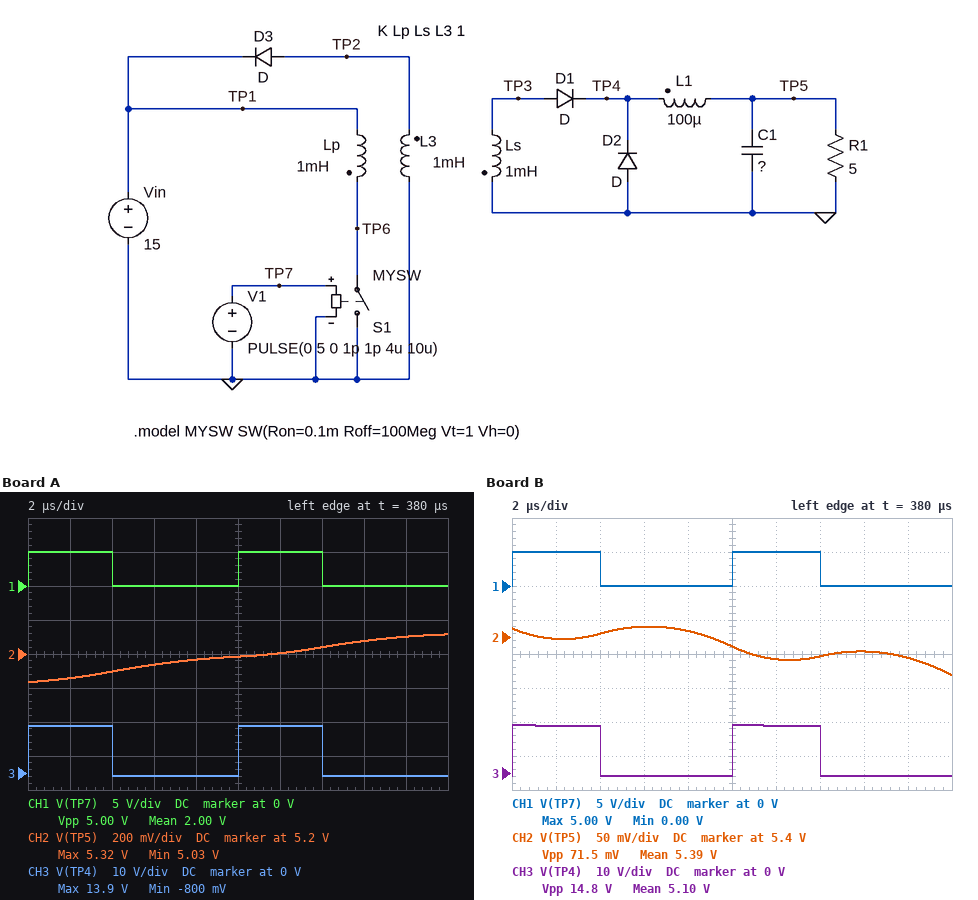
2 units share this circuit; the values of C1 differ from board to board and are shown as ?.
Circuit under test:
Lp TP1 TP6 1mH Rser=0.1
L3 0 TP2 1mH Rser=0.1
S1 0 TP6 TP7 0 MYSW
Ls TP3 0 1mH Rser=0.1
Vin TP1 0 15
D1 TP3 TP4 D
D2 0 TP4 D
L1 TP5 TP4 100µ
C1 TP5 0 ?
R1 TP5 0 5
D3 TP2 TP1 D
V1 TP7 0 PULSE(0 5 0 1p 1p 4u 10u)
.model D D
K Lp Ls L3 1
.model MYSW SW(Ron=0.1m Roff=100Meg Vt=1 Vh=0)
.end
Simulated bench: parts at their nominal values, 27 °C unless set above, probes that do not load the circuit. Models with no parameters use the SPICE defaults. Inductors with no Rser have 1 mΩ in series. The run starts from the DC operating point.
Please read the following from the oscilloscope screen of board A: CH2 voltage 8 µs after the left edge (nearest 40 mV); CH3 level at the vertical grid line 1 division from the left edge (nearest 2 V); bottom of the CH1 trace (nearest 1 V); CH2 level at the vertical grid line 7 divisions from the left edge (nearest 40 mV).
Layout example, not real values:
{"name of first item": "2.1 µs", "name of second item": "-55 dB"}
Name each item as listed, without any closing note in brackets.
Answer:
{"CH2 voltage 8 µs after the left edge": "5.16 V", "CH3 level at the vertical grid line 1 division from the left edge": "14 V", "bottom of the CH1 trace": "0 V", "CH2 level at the vertical grid line 7 divisions from the left edge": "5.24 V"}
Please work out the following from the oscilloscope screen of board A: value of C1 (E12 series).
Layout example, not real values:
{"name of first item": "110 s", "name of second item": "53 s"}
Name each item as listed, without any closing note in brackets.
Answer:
{"value of C1": "22 µF"}
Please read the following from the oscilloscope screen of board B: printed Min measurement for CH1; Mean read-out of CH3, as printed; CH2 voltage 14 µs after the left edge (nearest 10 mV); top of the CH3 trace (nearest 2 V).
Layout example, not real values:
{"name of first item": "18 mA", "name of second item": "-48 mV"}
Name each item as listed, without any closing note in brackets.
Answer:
{"printed Min measurement for CH1": "0.00 V", "Mean read-out of CH3, as printed": "5.10 V", "CH2 voltage 14 µs after the left edge": "5.37 V", "top of the CH3 trace": "14 V"}
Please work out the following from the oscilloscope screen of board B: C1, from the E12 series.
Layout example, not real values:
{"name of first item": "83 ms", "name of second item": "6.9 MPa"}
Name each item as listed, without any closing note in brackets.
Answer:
{"C1, from the E12 series": "15 µF"}
